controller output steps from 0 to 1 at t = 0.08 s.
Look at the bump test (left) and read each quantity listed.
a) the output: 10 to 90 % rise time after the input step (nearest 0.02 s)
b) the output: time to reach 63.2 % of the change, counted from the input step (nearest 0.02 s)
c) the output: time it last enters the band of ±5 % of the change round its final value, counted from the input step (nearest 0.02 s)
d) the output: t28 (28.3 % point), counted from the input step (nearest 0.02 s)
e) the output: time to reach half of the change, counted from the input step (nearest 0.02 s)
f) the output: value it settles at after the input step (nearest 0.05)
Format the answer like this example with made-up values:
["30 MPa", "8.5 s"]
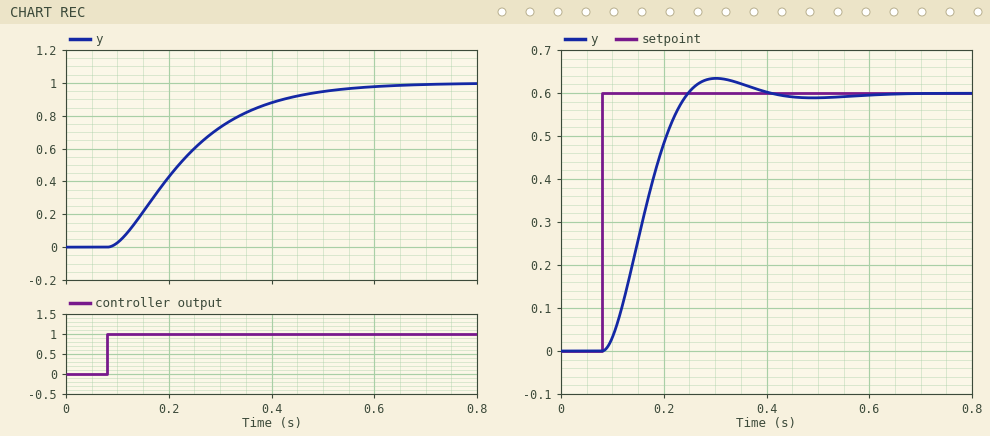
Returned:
["0.30 s", "0.18 s", "0.42 s", "0.08 s", "0.14 s", "1.00"]
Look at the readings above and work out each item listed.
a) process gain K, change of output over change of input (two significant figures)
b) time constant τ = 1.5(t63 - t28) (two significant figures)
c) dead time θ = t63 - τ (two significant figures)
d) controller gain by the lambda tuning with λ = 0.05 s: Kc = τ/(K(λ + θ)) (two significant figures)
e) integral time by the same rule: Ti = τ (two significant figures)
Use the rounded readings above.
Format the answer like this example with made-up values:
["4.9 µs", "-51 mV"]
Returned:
["1.0", "0.15 s", "0.030 s", "1.9", "0.15 s"]
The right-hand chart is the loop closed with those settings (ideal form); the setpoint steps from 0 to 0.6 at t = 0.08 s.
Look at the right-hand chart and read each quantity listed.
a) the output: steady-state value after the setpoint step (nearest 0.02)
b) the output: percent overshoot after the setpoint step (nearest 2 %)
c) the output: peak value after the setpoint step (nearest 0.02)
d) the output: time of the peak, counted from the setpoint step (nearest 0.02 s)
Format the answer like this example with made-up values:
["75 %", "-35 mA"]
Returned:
["0.60", "6 %", "0.64", "0.22 s"]
